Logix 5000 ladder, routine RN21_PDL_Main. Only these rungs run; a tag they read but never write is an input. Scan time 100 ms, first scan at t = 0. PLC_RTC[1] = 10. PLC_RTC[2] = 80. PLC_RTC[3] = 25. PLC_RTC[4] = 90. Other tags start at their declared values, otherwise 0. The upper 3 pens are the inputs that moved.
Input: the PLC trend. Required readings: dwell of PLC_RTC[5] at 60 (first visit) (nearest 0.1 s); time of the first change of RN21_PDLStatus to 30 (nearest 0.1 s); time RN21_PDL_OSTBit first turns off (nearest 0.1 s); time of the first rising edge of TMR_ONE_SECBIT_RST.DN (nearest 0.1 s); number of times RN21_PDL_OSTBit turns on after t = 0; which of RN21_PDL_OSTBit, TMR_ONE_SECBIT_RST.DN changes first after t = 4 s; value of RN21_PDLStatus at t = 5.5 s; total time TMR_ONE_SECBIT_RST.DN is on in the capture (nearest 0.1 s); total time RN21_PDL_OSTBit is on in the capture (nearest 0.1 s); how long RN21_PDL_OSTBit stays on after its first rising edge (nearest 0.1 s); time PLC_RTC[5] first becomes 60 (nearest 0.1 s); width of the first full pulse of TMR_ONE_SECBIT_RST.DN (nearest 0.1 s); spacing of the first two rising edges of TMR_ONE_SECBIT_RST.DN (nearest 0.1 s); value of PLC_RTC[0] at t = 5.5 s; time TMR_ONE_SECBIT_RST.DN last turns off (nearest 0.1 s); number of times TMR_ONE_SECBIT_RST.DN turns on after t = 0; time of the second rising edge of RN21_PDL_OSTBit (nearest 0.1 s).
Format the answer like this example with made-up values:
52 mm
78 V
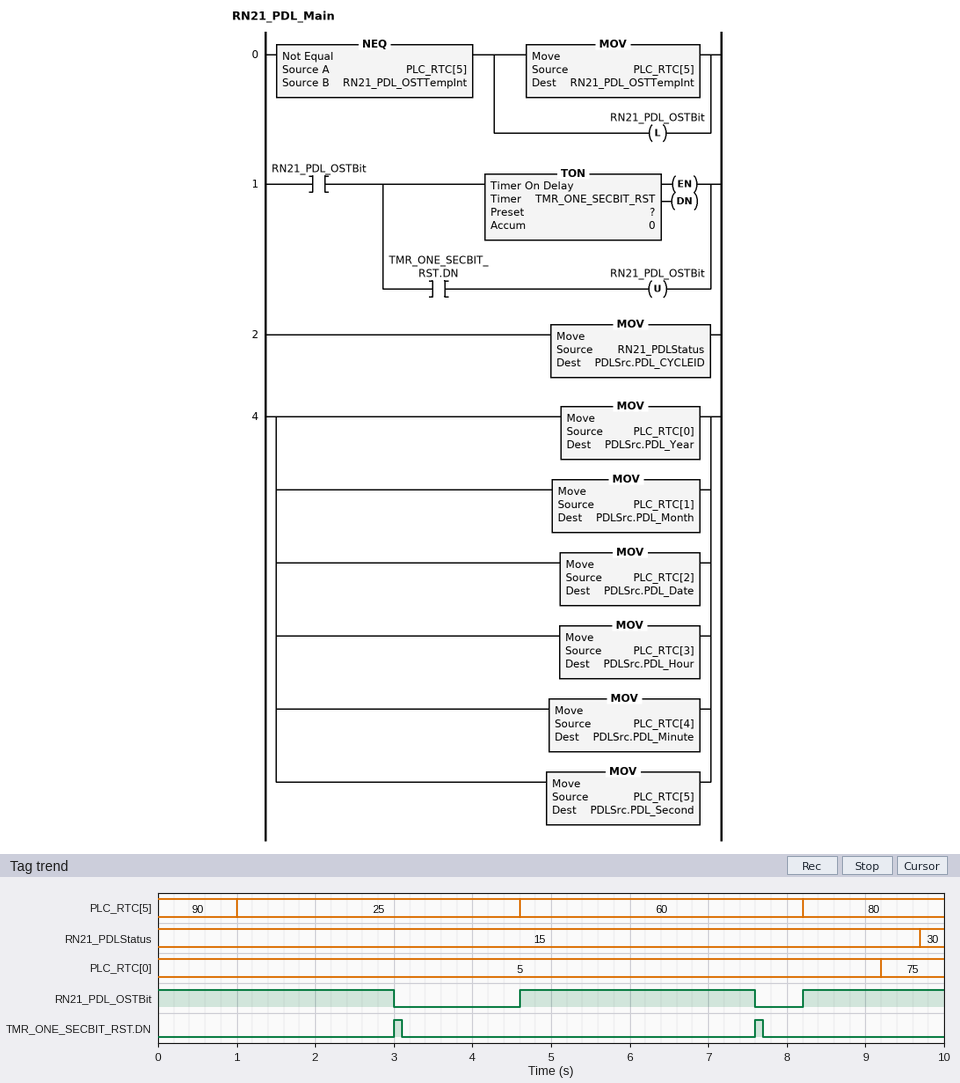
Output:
3.6 s
9.7 s
3.0 s
3.0 s
2
RN21_PDL_OSTBit
15
0.2 s
7.8 s
3.0 s
4.6 s
0.1 s
4.6 s
5
7.7 s
2
8.2 s
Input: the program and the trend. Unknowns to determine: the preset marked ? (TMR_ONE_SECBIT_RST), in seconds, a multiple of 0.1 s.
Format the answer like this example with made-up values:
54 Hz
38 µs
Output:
3.0 s
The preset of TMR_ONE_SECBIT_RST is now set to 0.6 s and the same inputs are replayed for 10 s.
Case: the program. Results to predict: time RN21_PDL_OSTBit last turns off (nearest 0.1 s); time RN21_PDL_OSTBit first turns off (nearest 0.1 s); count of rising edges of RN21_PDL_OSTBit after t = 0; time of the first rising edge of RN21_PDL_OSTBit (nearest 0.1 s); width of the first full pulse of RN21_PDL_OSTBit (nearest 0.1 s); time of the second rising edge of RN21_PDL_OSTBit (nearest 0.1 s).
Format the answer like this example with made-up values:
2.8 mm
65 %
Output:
8.8 s
0.6 s
3
1.0 s
0.6 s
4.6 s
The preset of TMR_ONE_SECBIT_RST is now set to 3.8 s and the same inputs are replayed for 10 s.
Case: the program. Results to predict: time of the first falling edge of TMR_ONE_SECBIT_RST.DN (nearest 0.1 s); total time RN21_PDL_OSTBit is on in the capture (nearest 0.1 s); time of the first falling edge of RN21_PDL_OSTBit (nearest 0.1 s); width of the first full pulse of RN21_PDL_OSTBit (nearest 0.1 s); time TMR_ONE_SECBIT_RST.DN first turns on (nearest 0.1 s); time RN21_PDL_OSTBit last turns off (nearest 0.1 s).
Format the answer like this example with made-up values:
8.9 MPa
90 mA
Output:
3.9 s
7.6 s
3.8 s
3.8 s
3.8 s
8.4 s
